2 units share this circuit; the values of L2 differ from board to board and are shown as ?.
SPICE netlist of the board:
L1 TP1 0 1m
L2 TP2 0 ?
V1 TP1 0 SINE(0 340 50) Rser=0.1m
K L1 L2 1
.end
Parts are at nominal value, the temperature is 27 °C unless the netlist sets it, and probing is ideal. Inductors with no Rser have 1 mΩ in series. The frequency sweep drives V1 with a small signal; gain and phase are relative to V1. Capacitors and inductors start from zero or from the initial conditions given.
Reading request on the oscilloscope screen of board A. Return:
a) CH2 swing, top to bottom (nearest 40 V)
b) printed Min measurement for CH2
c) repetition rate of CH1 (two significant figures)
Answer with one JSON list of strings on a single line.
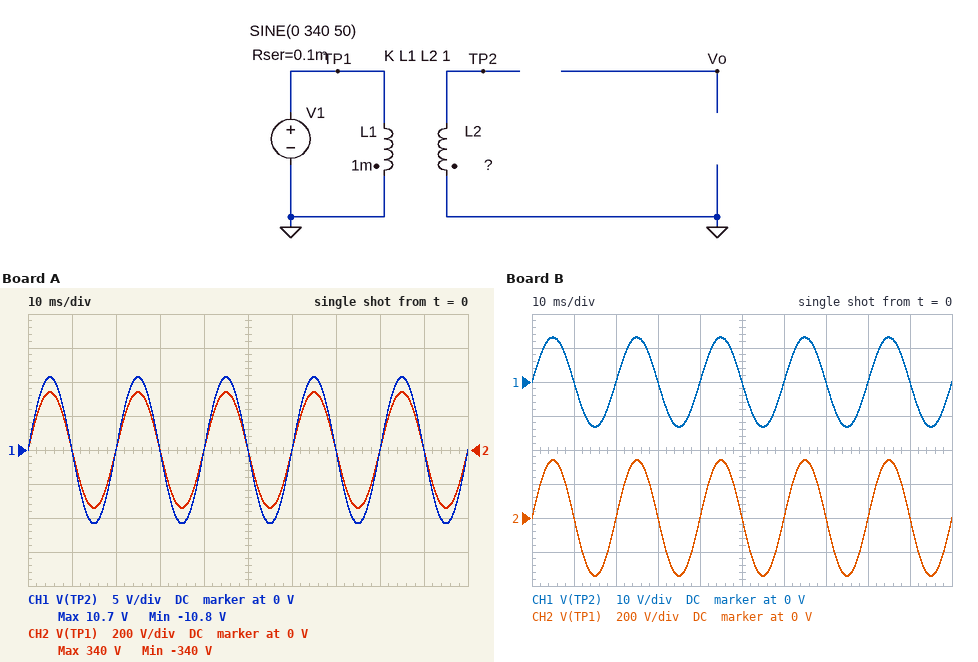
["680 V", "-340 V", "50 Hz"]
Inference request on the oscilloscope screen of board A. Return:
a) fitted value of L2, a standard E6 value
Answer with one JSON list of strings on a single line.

["1 µH"]
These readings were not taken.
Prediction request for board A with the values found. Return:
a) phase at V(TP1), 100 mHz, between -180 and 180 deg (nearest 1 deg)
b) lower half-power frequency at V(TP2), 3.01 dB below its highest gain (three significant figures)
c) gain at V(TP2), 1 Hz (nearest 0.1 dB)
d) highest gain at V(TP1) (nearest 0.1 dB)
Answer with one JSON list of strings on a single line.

["2 deg", "175 mHz", "-30.1 dB", "0 dB"]
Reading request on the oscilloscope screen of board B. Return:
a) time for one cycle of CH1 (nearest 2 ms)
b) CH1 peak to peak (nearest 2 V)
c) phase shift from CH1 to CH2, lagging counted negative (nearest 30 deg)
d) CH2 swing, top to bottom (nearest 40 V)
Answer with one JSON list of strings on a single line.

["20 ms", "26 V", "0 deg", "680 V"]
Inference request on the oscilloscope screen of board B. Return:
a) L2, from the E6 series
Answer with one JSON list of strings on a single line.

["1.5 µH"]
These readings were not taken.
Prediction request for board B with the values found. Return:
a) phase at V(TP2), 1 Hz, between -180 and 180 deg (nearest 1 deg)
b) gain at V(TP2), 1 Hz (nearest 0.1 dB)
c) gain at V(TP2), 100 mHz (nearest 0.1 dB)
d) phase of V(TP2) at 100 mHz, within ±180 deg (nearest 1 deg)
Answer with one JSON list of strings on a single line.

["10 deg", "-28.4 dB", "-34.3 dB", "60 deg"]
